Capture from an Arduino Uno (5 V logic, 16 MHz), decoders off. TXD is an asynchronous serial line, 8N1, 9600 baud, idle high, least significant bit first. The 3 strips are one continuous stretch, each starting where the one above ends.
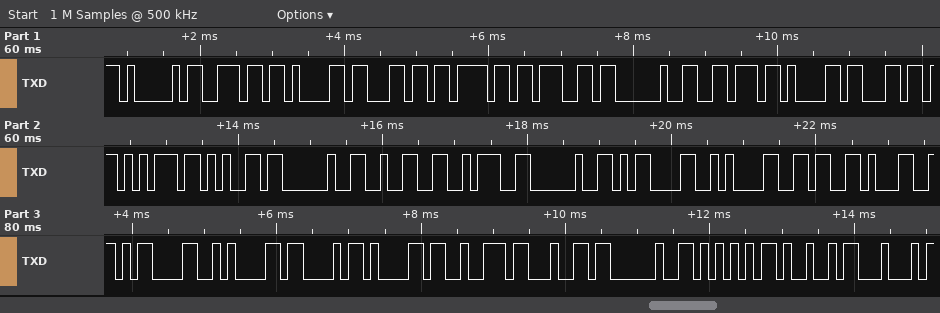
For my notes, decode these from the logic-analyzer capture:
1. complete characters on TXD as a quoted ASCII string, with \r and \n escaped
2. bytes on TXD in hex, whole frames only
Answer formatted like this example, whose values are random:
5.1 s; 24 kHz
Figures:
"Analog value 2: \r\n61\r\nCard UID"; 41 6E 61 6C 6F 67 20 76 61 6C 75 65 20 32 3A 20 0D 0A 36 31 0D 0A 43 61 72 64 20 55 49 44
